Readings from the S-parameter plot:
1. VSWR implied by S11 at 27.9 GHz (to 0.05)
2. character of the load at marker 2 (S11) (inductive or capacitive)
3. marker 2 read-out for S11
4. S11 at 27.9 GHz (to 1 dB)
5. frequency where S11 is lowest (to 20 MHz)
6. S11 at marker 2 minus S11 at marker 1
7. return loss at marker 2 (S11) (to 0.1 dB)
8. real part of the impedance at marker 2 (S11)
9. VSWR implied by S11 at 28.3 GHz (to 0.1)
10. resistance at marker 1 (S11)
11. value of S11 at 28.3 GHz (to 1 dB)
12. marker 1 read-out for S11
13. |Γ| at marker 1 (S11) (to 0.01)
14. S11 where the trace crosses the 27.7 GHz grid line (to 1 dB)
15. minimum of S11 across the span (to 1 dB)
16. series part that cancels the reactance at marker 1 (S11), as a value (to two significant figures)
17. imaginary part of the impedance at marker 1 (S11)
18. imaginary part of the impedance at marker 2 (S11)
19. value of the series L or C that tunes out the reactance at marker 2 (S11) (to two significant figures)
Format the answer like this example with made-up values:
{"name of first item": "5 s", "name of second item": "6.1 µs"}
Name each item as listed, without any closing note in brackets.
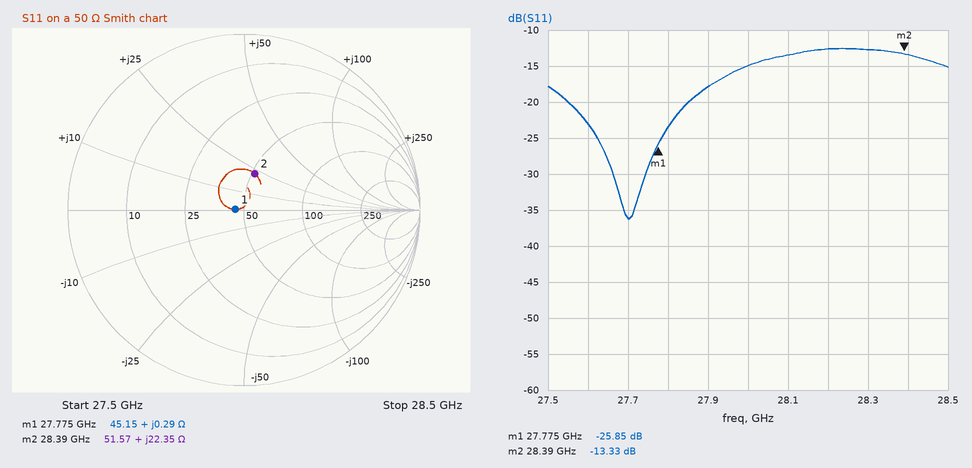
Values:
{"VSWR implied by S11 at 27.9 GHz": "1.30", "character of the load at marker 2 (S11)": "inductive", "marker 2 read-out for S11": "-13.33 dB", "S11 at 27.9 GHz": "-18 dB", "frequency where S11 is lowest": "27.70 GHz", "S11 at marker 2 minus S11 at marker 1": "12.52 dB", "return loss at marker 2 (S11)": "13.3 dB", "real part of the impedance at marker 2": "51.57 Ω", "VSWR implied by S11 at 28.3 GHz": "1.6", "resistance at marker 1": "45.15 Ω", "value of S11 at 28.3 GHz": "-13 dB", "marker 1 read-out for S11": "-25.85 dB", "|Γ| at marker 1 (S11)": "0.05", "S11 where the trace crosses the 27.7 GHz grid line": "-36 dB", "minimum of S11 across the span": "-36 dB", "series part that cancels the reactance at marker 1 (S11), as a value": "20 pF", "imaginary part of the impedance at marker 1": "+0.29 Ω", "imaginary part of the impedance at marker 2": "+22.35 Ω", "value of the series L or C that tunes out the reactance at marker 2 (S11)": "250 fF"}
